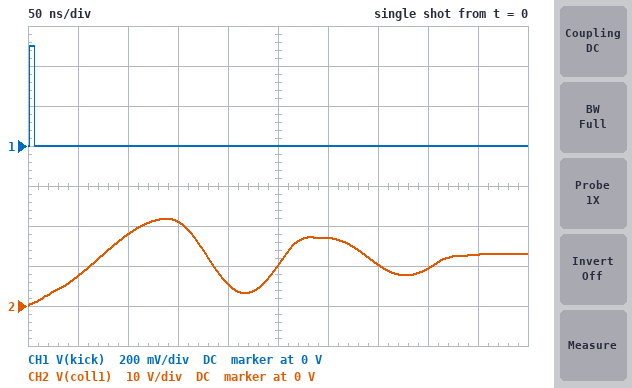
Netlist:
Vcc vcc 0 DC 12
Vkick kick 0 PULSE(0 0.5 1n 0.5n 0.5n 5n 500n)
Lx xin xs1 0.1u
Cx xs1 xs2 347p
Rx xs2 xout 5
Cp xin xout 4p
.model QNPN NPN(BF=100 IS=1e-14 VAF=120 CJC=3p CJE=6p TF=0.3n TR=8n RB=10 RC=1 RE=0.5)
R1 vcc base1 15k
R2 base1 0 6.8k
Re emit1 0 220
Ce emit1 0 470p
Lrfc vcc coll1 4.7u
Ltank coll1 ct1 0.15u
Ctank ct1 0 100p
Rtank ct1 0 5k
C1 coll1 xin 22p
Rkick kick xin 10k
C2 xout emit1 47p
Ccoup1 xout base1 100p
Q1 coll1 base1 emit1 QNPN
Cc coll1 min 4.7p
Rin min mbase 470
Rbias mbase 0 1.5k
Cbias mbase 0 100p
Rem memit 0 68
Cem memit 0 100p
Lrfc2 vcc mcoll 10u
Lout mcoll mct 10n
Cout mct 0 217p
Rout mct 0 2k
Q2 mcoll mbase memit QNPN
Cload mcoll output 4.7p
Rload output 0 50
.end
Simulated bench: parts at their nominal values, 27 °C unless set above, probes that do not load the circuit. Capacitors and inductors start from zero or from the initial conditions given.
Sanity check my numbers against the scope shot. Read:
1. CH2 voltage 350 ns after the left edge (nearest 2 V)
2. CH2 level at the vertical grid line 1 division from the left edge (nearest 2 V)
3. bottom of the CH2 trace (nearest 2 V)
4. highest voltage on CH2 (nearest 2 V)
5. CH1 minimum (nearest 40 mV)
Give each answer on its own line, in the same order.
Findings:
10 V
8 V
0 V
22 V
0 V
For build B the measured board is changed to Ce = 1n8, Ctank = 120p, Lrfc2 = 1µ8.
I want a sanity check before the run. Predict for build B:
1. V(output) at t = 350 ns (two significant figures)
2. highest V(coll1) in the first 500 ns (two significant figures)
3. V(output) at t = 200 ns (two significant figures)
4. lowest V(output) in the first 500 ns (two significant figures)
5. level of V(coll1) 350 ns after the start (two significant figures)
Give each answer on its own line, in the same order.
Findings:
-93 mV
22 V
-54 mV
-130 mV
20 V
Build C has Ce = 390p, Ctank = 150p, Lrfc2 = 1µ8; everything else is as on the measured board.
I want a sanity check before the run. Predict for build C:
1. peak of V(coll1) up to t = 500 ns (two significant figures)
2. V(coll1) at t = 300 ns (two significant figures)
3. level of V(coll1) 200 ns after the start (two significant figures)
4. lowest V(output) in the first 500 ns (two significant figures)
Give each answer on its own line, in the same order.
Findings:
22 V
16 V
9.1 V
-130 mV
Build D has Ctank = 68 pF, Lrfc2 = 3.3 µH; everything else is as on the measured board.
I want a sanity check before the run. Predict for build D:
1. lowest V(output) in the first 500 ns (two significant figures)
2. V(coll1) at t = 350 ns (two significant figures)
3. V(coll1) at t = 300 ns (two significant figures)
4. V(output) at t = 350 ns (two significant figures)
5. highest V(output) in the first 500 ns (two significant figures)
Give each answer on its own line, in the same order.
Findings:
-89 mV
8.6 V
13 V
21 mV
99 mV
